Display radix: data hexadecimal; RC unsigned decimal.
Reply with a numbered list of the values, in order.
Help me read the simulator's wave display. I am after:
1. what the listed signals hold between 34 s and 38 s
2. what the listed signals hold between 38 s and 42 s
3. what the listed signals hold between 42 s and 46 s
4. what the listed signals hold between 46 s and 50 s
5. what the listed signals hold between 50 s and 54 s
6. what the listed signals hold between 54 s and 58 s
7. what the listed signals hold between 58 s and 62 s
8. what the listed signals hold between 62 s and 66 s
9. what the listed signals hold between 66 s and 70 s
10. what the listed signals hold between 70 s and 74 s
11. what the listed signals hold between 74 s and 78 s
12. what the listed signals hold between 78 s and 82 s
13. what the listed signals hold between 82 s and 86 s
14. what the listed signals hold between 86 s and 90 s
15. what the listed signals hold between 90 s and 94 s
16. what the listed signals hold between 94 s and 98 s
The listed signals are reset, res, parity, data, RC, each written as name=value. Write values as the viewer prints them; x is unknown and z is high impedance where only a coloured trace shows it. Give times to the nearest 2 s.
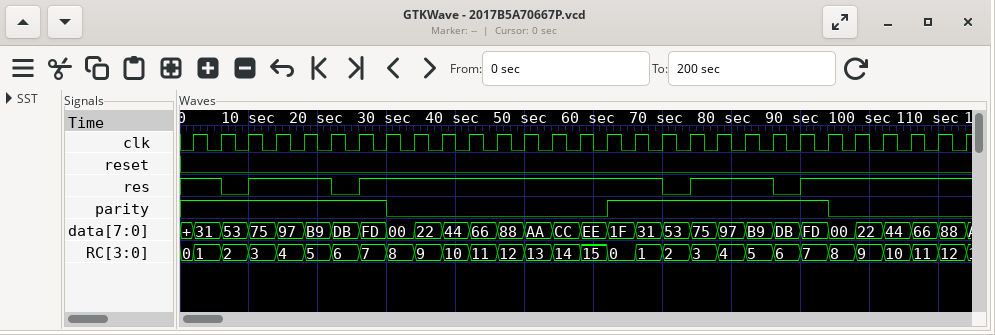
1. reset=0, res=1, parity=0, data=22, RC=9
2. reset=0, res=1, parity=0, data=44, RC=10
3. reset=0, res=1, parity=0, data=66, RC=11
4. reset=0, res=1, parity=0, data=88, RC=12
5. reset=0, res=1, parity=0, data=AA, RC=13
6. reset=0, res=1, parity=0, data=CC, RC=14
7. reset=0, res=1, parity=0, data=EE, RC=15
8. reset=0, res=1, parity=1, data=1F, RC=0
9. reset=0, res=1, parity=1, data=31, RC=1
10. reset=0, res=0, parity=1, data=53, RC=2
11. reset=0, res=1, parity=1, data=75, RC=3
12. reset=0, res=1, parity=1, data=97, RC=4
13. reset=0, res=1, parity=1, data=B9, RC=5
14. reset=0, res=0, parity=1, data=DB, RC=6
15. reset=0, res=1, parity=1, data=FD, RC=7
16. reset=0, res=1, parity=0, data=00, RC=8
